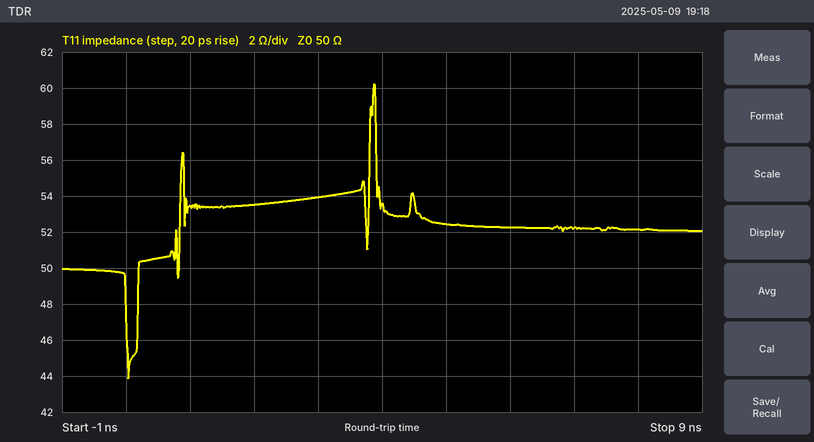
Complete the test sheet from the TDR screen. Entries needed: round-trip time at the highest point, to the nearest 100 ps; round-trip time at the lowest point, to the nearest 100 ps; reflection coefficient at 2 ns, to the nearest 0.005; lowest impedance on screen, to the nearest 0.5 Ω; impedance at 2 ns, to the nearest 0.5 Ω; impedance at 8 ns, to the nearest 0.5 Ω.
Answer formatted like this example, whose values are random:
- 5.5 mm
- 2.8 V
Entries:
- 3.9 ns
- 0.0 ns
- +0.035
- 44.0 Ω
- 53.5 Ω
- 52.0 Ω
